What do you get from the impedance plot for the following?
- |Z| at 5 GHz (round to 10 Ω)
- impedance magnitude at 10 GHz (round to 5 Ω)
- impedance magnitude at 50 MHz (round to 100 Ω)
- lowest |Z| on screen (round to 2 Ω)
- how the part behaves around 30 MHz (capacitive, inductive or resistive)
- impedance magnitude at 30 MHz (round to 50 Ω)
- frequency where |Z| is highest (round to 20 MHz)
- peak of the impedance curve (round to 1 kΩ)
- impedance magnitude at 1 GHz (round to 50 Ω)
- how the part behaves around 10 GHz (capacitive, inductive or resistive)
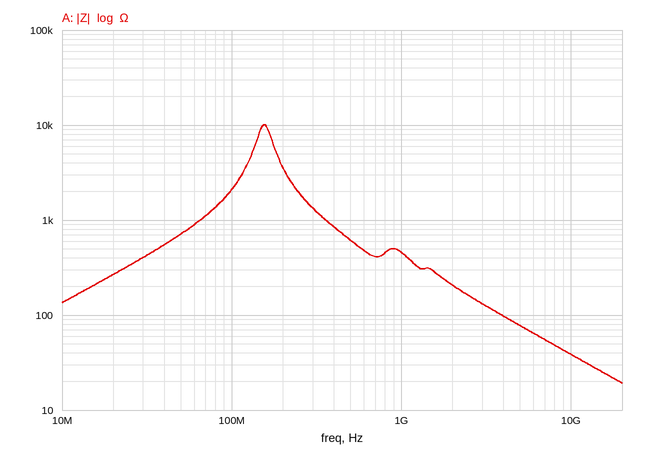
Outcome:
80 Ω
40 Ω
700 Ω
20 Ω
inductive
400 Ω
160 MHz
10 kΩ
450 Ω
capacitive
